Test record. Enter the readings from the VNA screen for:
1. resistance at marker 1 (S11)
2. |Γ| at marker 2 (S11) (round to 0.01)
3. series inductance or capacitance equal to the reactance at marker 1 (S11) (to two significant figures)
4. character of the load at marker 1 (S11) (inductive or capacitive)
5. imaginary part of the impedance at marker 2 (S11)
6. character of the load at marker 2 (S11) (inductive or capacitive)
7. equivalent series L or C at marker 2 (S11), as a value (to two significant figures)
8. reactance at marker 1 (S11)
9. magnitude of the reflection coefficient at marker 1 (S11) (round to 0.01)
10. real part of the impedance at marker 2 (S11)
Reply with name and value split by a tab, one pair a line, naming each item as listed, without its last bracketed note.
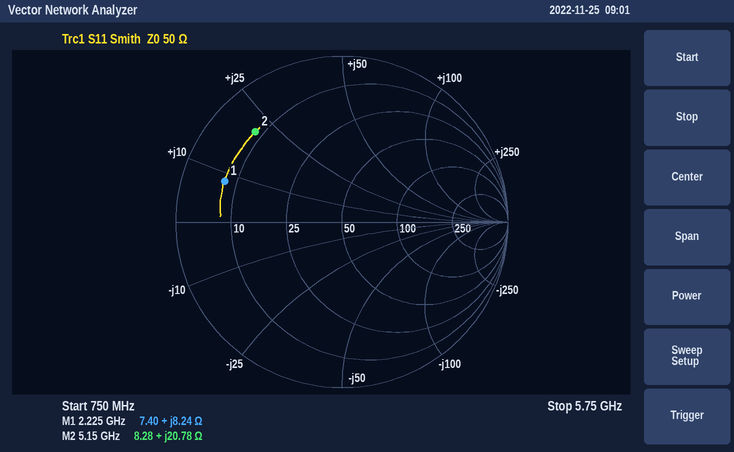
resistance at marker 1	7.40 Ω
|Γ| at marker 2 (S11)	0.75
series inductance or capacitance equal to the reactance at marker 1 (S11)	590 pH
character of the load at marker 1 (S11)	inductive
imaginary part of the impedance at marker 2	+20.78 Ω
character of the load at marker 2 (S11)	inductive
equivalent series L or C at marker 2 (S11), as a value	640 pH
reactance at marker 1	+8.24 Ω
magnitude of the reflection coefficient at marker 1 (S11)	0.75
real part of the impedance at marker 2	8.28 Ω
